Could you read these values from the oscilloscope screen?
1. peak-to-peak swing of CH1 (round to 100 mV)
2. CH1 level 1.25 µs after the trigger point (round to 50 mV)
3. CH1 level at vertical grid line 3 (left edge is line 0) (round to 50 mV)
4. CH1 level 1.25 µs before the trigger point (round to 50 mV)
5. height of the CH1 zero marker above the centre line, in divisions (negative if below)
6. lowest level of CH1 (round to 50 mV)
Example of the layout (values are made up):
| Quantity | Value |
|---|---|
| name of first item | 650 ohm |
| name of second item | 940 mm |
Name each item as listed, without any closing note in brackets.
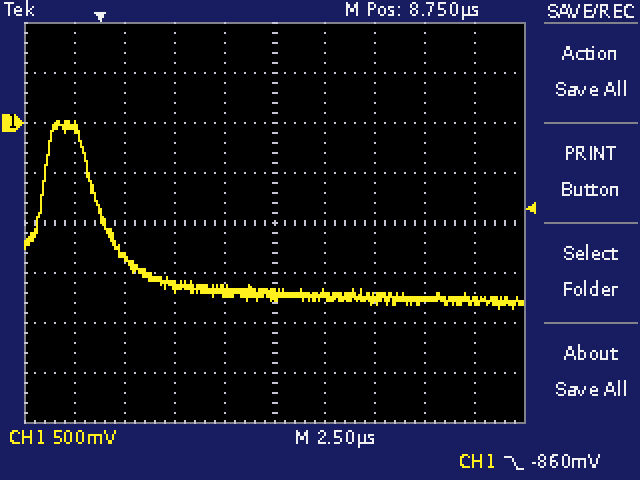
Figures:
| Quantity | Value |
|---|---|
| peak-to-peak swing of CH1 | 1.90 V |
| CH1 level 1.25 µs after the trigger point | -1.35 V |
| CH1 level at vertical grid line 3 (left edge is line 0) | -1.65 V |
| CH1 level 1.25 µs before the trigger point | -50 mV |
| height of the CH1 zero marker above the centre line, in divisions | +2.0 div |
| lowest level of CH1 | -1.85 V |
